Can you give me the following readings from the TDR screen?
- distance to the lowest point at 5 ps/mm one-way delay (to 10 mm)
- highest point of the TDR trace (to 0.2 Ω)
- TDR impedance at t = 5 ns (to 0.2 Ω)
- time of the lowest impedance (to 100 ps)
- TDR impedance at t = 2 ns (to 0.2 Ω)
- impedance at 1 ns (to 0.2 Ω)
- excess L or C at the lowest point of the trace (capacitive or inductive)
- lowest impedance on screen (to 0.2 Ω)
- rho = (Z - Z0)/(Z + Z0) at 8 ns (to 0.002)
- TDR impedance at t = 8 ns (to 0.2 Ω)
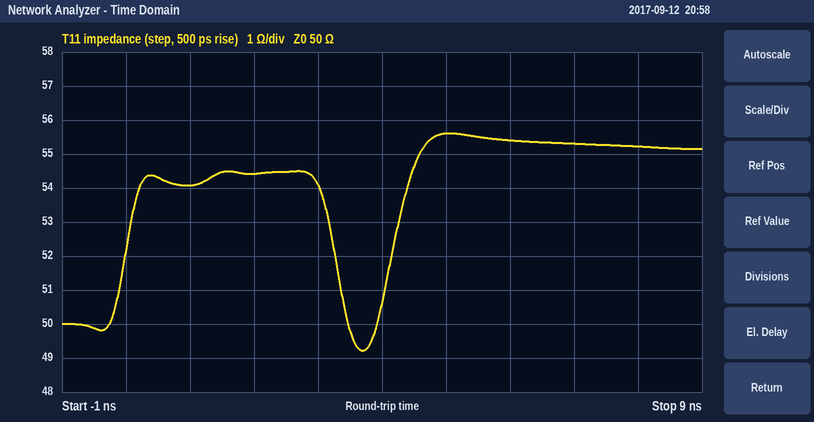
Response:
370 mm
55.6 Ω
55.6 Ω
3.7 ns
54.4 Ω
54.0 Ω
capacitive
49.2 Ω
+0.050
55.2 Ω
